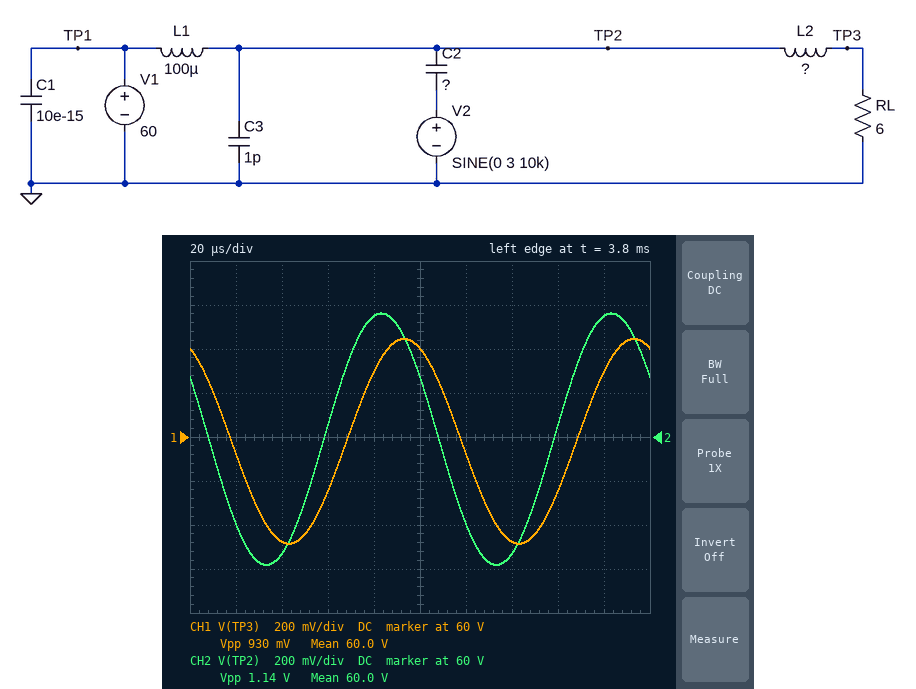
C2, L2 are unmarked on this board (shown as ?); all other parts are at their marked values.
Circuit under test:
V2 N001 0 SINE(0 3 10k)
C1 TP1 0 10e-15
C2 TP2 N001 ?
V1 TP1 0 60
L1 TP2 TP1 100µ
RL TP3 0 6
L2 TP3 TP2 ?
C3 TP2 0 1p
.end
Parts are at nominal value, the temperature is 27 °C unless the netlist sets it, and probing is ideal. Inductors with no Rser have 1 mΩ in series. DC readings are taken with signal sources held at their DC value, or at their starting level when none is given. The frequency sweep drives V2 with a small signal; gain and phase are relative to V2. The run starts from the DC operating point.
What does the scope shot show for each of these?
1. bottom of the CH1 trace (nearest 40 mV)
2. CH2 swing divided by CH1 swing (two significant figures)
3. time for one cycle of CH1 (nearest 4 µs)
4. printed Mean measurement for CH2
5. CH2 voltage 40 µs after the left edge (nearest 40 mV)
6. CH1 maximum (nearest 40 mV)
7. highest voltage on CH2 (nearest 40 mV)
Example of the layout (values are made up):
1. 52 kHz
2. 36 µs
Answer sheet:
1. 59.52 V
2. 1.2
3. 100 µs
4. 60.0 V
5. 59.48 V
6. 60.44 V
7. 60.56 V
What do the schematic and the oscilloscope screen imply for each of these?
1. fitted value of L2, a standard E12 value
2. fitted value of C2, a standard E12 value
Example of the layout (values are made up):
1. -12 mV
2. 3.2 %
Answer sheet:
1. 68 µH
2. 680 nF
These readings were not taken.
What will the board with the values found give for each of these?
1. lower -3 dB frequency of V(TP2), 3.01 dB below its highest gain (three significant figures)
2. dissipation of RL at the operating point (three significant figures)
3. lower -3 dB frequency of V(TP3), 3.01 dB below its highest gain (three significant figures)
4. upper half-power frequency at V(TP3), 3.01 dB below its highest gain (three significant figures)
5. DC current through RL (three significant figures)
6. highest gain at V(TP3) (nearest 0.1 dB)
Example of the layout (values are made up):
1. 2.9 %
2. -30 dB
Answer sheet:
1. 26.5 kHz
2. 600 W
3. 25.8 kHz
4. 33.9 kHz
5. 10.0 A
6. 4.7 dB
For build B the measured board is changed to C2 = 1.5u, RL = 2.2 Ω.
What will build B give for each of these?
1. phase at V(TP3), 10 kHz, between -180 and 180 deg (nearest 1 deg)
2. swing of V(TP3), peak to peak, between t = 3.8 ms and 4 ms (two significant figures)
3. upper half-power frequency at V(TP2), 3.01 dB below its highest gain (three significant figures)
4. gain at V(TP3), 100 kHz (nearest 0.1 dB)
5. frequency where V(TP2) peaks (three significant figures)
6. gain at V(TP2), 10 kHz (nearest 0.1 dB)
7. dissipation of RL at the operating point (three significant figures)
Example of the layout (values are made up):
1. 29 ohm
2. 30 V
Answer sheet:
1. 96 deg
2. 970 mV
3. 22.1 kHz
4. -25.4 dB
5. 20.4 kHz
6. -9.1 dB
7. 1.63 kW
